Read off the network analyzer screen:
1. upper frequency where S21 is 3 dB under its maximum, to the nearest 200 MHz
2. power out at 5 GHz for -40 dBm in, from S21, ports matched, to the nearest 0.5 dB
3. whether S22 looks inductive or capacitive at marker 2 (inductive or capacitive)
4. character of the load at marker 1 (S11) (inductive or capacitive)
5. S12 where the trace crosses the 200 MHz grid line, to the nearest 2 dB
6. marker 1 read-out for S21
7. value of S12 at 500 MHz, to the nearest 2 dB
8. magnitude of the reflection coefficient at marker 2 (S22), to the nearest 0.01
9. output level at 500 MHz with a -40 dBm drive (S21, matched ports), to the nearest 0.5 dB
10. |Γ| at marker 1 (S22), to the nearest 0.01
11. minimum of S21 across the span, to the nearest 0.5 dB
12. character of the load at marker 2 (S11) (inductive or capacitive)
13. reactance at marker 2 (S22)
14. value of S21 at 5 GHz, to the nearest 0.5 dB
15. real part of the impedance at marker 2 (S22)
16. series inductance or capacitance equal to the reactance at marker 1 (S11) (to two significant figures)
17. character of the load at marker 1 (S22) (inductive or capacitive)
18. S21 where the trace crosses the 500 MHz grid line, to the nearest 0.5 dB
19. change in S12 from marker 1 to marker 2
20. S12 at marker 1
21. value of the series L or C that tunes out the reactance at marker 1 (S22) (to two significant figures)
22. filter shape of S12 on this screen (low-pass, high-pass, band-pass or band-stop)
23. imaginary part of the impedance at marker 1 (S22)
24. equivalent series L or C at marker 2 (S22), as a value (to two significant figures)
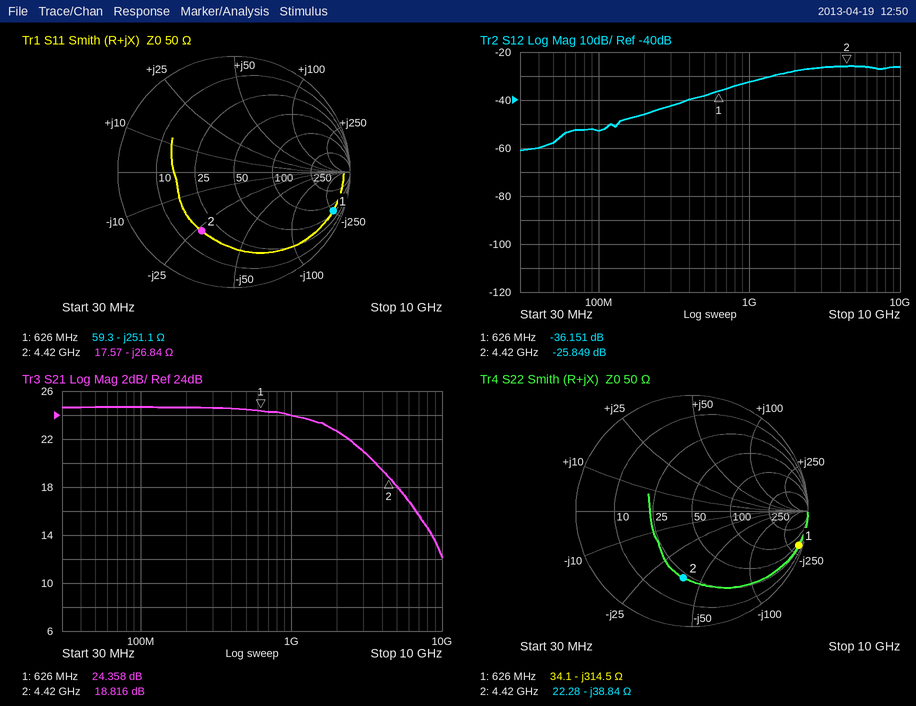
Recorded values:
2.6 GHz
-22.0 dBm
capacitive
capacitive
-46 dB
24.358 dB
-38 dB
0.58
-15.5 dBm
0.97
12.0 dB
capacitive
-38.84 Ω
18.0 dB
22.28 Ω
1.0 pF
capacitive
24.5 dB
10.302 dB
-36.151 dB
80 nH
high-pass
-314.5 Ω
930 fF
